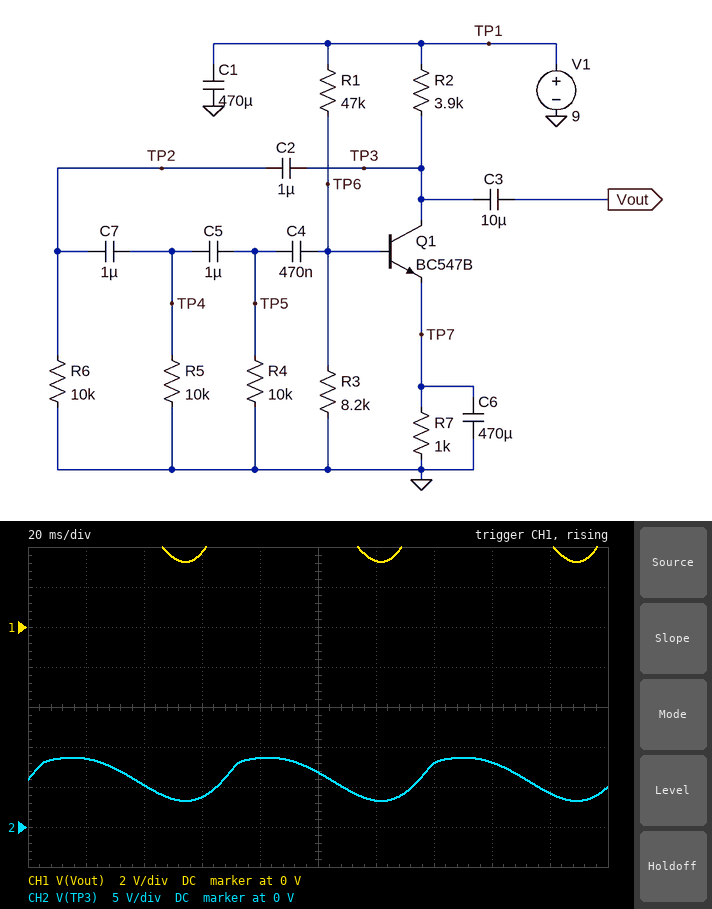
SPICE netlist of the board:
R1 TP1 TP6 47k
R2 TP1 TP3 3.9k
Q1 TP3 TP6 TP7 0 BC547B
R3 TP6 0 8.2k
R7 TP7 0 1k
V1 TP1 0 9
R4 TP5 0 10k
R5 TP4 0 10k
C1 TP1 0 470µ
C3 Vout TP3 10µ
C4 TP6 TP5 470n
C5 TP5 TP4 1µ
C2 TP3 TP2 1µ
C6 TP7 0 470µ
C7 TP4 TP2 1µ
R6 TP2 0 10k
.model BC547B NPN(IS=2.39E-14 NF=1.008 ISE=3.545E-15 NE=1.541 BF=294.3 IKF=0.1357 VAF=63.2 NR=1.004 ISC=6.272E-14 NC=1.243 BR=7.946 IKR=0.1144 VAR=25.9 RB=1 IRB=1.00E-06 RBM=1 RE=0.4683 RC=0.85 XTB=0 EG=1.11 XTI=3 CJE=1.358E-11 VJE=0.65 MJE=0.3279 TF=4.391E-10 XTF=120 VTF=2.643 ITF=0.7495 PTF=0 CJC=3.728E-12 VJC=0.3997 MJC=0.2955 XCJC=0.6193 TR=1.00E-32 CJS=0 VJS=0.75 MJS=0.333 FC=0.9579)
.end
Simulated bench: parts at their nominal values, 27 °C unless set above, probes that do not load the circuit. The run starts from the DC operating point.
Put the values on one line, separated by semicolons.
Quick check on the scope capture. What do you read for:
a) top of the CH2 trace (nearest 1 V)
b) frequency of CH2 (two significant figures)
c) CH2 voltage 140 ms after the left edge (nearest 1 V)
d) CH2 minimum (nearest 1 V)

9 V; 15 Hz; 8 V; 3 V
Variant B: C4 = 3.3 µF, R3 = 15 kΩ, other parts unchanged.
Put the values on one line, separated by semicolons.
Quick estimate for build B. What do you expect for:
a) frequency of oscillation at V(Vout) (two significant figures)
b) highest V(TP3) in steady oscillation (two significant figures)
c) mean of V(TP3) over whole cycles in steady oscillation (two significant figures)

9.4 Hz; 6.0 V; 3.5 V
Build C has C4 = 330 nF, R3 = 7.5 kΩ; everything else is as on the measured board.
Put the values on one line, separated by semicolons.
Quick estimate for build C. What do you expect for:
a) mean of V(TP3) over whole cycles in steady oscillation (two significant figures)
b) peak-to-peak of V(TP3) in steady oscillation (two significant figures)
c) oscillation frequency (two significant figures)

6.6 V; 4.4 V; 17 Hz
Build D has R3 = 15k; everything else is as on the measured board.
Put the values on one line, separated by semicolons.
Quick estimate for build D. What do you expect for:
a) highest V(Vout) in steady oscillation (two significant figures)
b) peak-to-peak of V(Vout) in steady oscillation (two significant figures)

5.6 V; 4.2 V
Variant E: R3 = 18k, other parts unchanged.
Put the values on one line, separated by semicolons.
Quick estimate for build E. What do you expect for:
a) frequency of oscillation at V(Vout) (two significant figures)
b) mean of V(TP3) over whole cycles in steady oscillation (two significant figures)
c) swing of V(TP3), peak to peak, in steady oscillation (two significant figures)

16 Hz; 2.2 V; 700 mV
